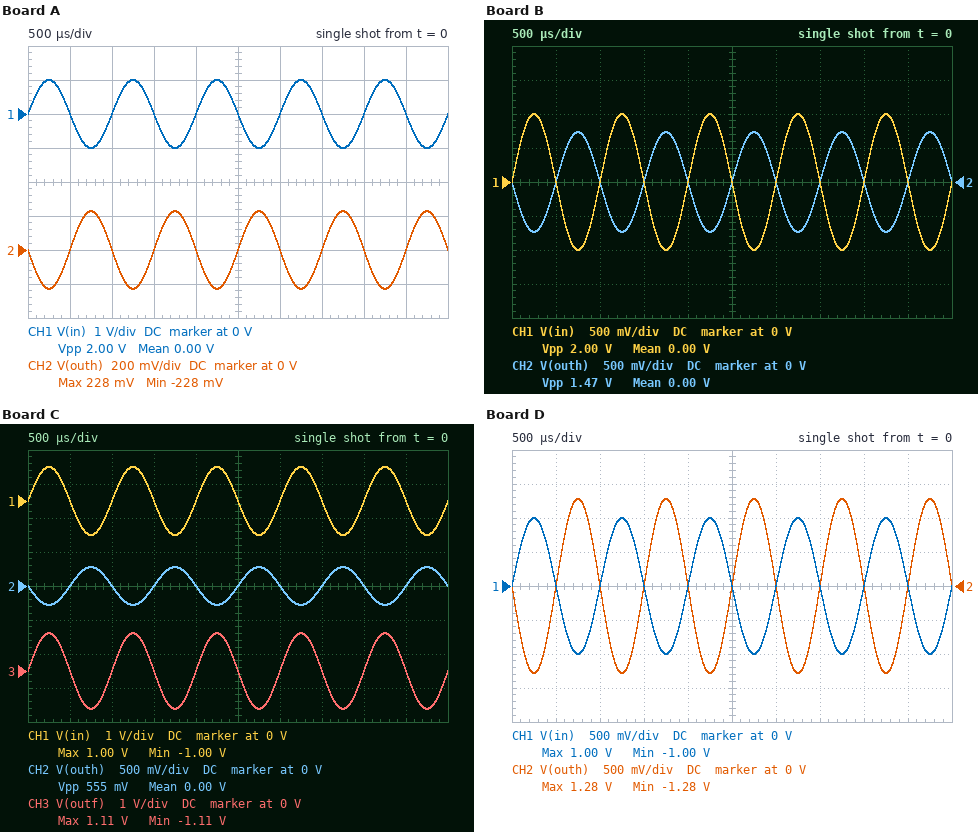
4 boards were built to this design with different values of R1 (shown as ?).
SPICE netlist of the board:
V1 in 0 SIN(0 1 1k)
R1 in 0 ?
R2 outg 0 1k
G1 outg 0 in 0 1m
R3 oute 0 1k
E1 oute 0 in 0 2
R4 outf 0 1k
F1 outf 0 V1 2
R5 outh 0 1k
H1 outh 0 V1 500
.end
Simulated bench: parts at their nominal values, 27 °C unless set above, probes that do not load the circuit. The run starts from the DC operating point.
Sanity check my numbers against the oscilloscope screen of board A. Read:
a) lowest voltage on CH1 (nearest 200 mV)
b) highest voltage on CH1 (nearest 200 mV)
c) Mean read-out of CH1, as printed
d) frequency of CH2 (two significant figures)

-1.0 V
1.0 V
0.00 V
1.0 kHz
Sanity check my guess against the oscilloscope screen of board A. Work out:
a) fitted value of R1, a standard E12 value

2.2 kΩ
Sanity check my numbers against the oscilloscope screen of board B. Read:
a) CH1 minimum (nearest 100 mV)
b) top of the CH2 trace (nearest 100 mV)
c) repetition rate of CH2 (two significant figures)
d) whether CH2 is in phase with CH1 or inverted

-1.0 V
700 mV
1.0 kHz
inverted
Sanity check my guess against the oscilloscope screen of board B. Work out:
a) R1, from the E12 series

680 Ω
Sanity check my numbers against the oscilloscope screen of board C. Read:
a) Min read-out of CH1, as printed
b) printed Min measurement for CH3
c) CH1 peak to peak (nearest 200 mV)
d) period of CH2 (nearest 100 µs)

-1.00 V
-1.11 V
2.0 V
1.0 ms
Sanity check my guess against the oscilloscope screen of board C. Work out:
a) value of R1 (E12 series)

1.8 kΩ
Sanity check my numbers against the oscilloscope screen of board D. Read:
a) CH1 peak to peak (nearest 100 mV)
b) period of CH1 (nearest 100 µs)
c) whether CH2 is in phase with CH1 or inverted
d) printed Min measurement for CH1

2.0 V
1.0 ms
inverted
-1.00 V
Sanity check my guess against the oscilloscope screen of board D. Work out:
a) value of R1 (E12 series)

390 Ω
